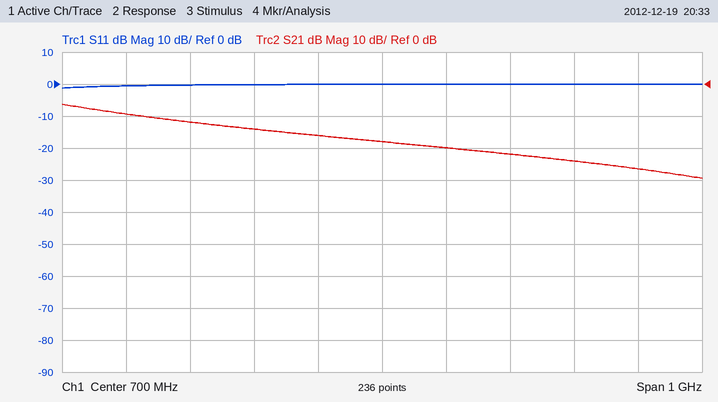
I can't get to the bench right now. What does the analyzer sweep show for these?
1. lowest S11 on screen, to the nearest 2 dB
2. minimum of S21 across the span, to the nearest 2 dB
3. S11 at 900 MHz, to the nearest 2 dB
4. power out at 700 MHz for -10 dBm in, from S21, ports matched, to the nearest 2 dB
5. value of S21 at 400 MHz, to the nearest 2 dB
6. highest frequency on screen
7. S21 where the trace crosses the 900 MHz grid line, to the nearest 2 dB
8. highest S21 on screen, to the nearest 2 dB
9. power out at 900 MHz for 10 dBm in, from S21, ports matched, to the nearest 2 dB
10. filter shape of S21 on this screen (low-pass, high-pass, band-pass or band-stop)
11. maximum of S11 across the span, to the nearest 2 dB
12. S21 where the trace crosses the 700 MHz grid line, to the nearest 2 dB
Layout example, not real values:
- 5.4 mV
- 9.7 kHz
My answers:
- -2 dB
- -30 dB
- 0 dB
- -28 dBm
- -12 dB
- 1.2 GHz
- -22 dB
- -6 dB
- -12 dBm
- low-pass
- 0 dB
- -18 dB
